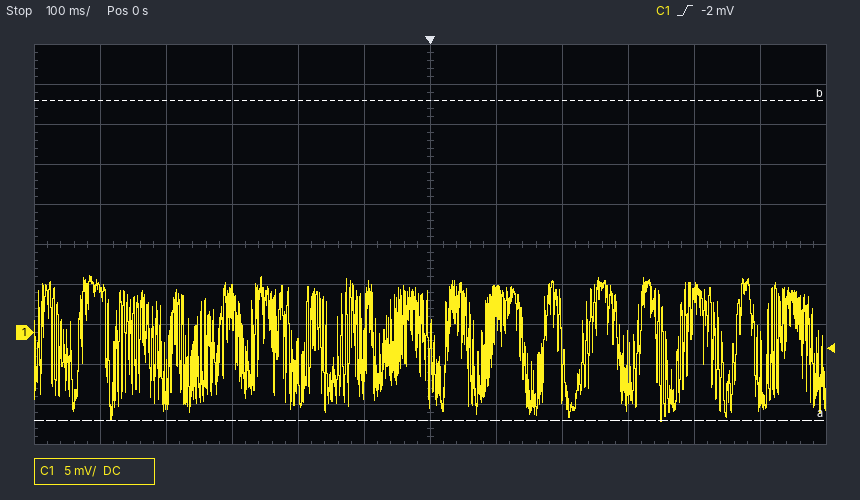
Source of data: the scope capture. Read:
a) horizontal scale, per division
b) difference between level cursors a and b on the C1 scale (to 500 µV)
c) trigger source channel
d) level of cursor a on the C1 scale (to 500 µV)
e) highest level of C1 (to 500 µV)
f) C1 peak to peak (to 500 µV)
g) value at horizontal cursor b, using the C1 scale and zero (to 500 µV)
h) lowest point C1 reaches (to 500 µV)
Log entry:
100 ms
40.0 mV
C1
-11.0 mV
7.0 mV
18.0 mV
29.0 mV
-11.0 mV
